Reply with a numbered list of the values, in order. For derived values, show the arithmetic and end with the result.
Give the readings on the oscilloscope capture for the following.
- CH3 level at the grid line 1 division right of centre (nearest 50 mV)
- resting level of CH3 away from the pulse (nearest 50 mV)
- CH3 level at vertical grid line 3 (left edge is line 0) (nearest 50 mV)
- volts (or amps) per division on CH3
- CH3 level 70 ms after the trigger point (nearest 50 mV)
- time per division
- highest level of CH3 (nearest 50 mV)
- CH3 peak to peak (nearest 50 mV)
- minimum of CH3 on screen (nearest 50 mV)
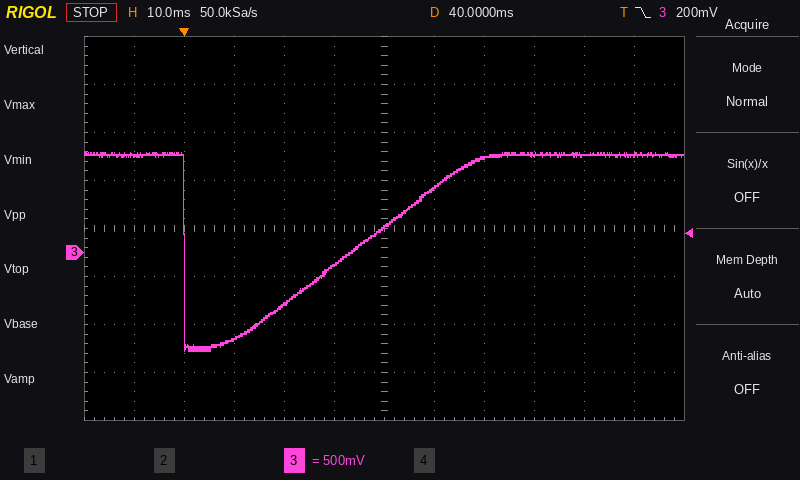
1. 650 mV
2. 1.00 V
3. -900 mV
4. 500 mV
5. 1.00 V
6. 10 ms
7. 1.05 V
8. 1.05 V − (-1.00 V) = 2.05 V
9. -1.00 V
